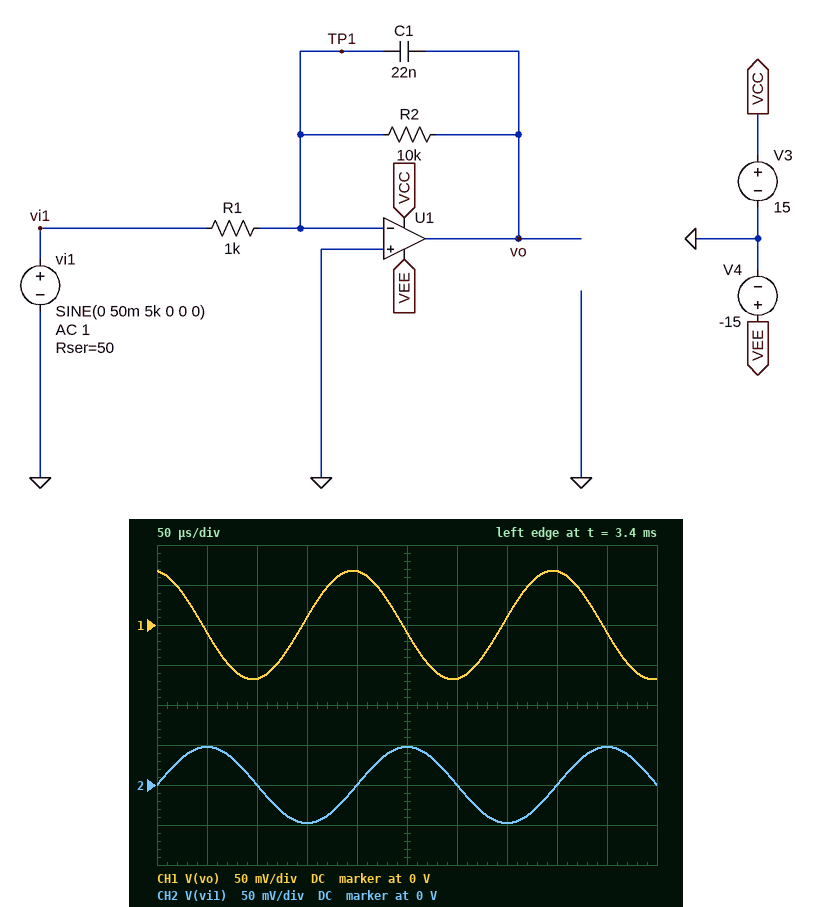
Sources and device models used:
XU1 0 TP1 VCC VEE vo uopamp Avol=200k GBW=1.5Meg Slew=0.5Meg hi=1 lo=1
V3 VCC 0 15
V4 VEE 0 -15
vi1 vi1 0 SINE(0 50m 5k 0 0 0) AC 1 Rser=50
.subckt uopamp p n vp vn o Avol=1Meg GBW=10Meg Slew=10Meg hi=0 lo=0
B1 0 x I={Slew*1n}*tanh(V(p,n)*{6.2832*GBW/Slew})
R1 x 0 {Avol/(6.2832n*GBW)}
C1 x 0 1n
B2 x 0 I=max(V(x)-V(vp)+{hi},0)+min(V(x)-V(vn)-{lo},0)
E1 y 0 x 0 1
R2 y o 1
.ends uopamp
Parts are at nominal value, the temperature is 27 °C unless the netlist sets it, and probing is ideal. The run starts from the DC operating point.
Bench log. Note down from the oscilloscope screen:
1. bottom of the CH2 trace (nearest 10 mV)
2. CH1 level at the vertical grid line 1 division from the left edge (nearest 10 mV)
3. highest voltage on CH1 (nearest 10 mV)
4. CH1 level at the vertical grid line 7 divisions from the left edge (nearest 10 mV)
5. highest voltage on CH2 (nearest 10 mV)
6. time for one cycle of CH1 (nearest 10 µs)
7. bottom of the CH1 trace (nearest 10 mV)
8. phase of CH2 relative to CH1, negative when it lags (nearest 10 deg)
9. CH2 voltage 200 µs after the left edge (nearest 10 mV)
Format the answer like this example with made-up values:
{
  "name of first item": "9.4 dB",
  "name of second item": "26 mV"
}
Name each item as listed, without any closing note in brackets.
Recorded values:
{
  "bottom of the CH2 trace": "-50 mV",
  "CH1 level at the vertical grid line 1 division from the left edge": "-10 mV",
  "highest voltage on CH1": "70 mV",
  "CH1 level at the vertical grid line 7 divisions from the left edge": "10 mV",
  "highest voltage on CH2": "50 mV",
  "time for one cycle of CH1": "200 µs",
  "bottom of the CH1 trace": "-70 mV",
  "phase of CH2 relative to CH1, negative when it lags": "-100 deg",
  "CH2 voltage 200 µs after the left edge": "0 V"
}
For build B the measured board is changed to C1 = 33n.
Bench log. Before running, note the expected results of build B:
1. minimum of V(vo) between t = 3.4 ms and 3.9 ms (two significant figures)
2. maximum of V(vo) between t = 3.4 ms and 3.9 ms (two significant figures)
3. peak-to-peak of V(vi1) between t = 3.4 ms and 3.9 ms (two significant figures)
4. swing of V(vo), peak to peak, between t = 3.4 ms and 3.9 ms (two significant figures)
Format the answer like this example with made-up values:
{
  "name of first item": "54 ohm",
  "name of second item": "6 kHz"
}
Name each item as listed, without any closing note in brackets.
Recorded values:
{
  "minimum of V(vo) between t = 3.4 ms and 3.9 ms": "-46 mV",
  "maximum of V(vo) between t = 3.4 ms and 3.9 ms": "46 mV",
  "peak-to-peak of V(vi1) between t = 3.4 ms and 3.9 ms": "95 mV",
  "swing of V(vo), peak to peak, between t = 3.4 ms and 3.9 ms": "91 mV"
}
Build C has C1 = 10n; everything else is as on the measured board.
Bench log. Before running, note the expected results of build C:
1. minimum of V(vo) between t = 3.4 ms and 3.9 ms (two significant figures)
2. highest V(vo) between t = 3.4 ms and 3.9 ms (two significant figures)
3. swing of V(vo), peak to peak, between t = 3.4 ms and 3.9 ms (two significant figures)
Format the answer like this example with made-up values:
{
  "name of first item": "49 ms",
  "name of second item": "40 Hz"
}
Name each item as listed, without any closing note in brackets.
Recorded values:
{
  "minimum of V(vo) between t = 3.4 ms and 3.9 ms": "-140 mV",
  "highest V(vo) between t = 3.4 ms and 3.9 ms": "140 mV",
  "swing of V(vo), peak to peak, between t = 3.4 ms and 3.9 ms": "290 mV"
}
